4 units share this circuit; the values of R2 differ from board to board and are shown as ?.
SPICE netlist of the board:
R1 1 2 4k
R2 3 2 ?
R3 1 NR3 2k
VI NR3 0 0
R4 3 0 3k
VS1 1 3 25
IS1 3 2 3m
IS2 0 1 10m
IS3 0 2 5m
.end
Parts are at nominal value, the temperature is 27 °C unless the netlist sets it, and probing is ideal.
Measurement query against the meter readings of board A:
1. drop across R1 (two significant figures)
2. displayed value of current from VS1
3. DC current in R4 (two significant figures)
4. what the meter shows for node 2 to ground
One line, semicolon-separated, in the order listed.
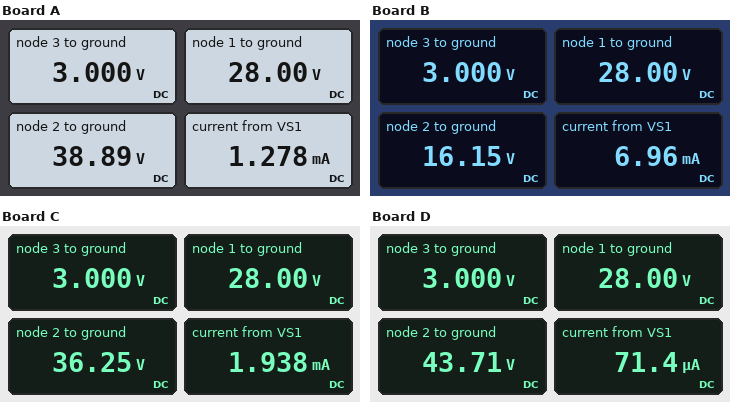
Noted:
11 V; 1.278 mA; 1.0 mA; 38.89 V
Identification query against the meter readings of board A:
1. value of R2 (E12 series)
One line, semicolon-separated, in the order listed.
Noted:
6.8 kΩ
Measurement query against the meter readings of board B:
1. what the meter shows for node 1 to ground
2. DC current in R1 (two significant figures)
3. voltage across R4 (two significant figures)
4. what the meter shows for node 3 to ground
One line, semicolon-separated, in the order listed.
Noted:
28.00 V; 3.0 mA; 3.0 V; 3.000 V
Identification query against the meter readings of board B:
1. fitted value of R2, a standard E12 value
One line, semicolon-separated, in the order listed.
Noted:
1.2 kΩ
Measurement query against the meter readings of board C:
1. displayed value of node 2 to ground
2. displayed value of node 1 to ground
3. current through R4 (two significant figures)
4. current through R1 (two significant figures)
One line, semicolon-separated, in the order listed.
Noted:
36.25 V; 28.00 V; 1.0 mA; 2.1 mA
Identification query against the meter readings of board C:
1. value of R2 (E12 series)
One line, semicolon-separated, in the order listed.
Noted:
5.6 kΩ
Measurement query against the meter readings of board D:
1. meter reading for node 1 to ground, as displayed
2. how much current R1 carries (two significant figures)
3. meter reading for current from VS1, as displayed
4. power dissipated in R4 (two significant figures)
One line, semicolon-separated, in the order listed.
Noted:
28.00 V; 3.9 mA; 71.4 µA; 3.0 mW
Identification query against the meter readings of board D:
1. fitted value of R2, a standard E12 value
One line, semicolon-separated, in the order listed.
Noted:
10 kΩ
